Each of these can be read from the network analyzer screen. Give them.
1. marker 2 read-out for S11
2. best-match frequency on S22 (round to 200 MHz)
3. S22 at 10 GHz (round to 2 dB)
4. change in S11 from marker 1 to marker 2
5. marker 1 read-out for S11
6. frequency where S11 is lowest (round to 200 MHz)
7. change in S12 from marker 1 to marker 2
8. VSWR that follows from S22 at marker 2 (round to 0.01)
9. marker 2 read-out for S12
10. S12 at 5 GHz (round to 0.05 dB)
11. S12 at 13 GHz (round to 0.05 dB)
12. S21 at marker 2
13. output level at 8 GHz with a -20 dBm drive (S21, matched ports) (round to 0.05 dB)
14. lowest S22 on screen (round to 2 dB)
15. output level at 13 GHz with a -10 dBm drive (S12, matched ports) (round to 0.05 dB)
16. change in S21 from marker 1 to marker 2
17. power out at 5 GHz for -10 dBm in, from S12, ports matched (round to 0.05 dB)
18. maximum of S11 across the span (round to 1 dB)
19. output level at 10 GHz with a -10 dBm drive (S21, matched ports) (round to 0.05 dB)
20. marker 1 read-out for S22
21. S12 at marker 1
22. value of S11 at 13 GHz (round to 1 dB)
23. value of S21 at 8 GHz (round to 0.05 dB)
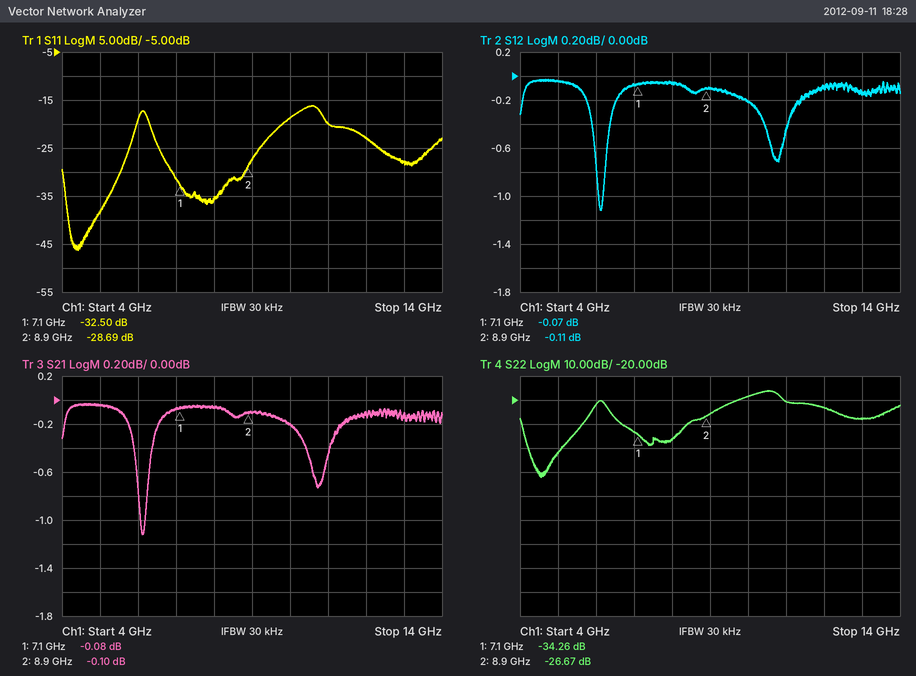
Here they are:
-28.69 dB
4.6 GHz
-18 dB
3.81 dB
-32.50 dB
4.4 GHz
-0.04 dB
1.10
-0.11 dB
-0.05 dB
-0.15 dB
-0.10 dB
-20.05 dBm
-52 dB
-10.15 dBm
-0.02 dB
-10.05 dBm
-16 dB
-10.20 dBm
-34.26 dB
-0.07 dB
-28 dB
-0.05 dB
